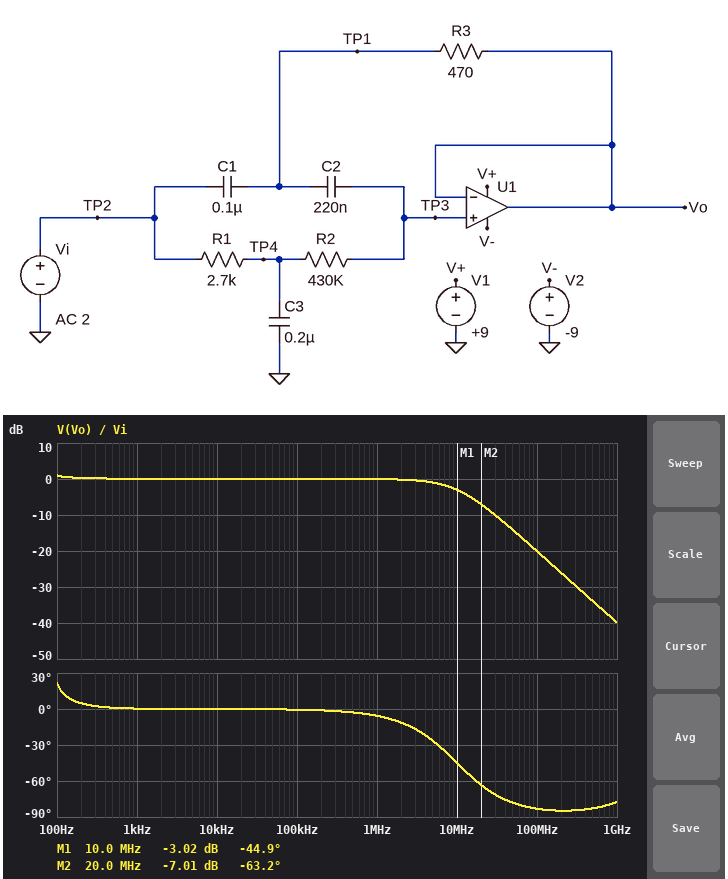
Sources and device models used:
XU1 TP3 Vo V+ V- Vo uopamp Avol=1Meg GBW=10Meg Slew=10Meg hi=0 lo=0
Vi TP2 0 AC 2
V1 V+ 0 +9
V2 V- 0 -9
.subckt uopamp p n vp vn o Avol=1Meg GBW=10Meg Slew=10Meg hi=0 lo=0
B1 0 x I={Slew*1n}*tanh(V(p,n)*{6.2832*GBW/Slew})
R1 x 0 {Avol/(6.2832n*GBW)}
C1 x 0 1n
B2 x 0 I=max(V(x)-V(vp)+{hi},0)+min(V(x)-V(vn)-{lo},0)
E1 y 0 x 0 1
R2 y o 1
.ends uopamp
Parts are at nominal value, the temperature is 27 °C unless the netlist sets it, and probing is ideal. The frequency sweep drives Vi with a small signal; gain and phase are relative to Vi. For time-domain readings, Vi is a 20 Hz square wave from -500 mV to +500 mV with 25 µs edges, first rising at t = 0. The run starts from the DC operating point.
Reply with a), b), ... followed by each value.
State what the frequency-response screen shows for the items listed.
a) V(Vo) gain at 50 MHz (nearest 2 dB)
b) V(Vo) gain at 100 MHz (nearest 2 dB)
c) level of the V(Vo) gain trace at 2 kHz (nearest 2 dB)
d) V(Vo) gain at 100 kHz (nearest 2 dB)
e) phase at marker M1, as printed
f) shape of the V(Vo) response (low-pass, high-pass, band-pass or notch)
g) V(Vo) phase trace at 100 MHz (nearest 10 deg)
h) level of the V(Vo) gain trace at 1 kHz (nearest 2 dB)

a) -14 dB
b) -20 dB
c) 0 dB
d) 0 dB
e) -44.9 deg
f) low-pass
g) -80 deg
h) 0 dB
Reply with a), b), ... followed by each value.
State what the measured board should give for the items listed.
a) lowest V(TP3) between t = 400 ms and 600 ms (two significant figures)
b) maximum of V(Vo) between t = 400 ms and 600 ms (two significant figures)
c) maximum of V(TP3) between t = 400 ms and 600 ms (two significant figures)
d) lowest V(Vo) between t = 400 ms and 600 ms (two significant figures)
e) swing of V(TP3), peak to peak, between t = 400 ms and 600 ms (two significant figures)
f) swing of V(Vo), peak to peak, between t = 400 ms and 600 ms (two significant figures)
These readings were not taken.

a) -640 mV
b) 640 mV
c) 640 mV
d) -640 mV
e) 1.3 V
f) 1.3 V
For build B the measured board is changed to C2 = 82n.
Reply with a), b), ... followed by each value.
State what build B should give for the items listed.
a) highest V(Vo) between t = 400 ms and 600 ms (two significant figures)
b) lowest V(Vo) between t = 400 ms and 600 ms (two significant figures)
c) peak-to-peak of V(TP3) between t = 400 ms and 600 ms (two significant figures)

a) 720 mV
b) -720 mV
c) 1.4 V
